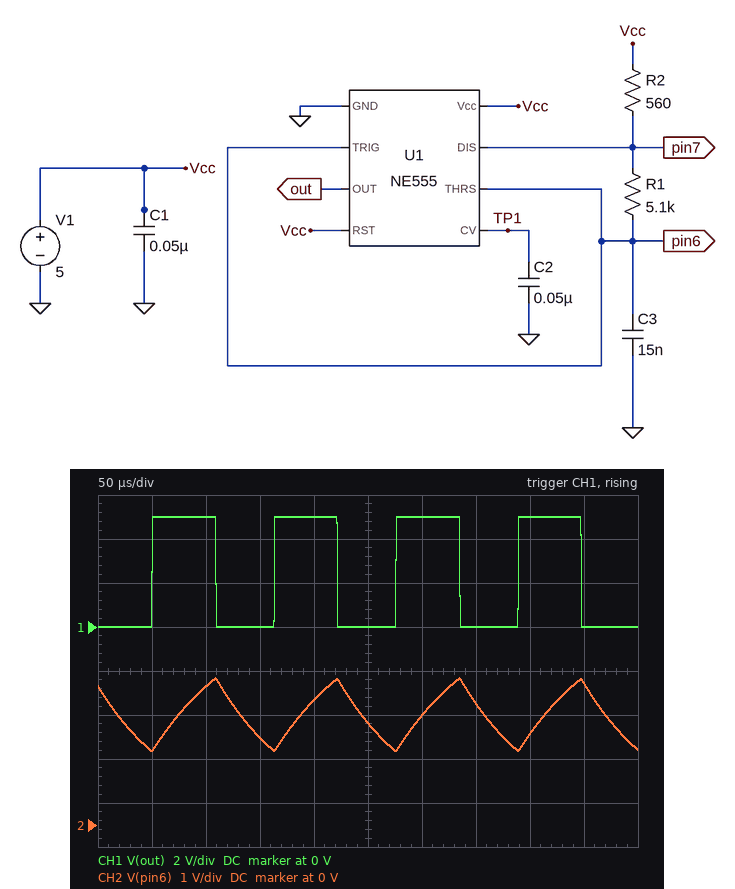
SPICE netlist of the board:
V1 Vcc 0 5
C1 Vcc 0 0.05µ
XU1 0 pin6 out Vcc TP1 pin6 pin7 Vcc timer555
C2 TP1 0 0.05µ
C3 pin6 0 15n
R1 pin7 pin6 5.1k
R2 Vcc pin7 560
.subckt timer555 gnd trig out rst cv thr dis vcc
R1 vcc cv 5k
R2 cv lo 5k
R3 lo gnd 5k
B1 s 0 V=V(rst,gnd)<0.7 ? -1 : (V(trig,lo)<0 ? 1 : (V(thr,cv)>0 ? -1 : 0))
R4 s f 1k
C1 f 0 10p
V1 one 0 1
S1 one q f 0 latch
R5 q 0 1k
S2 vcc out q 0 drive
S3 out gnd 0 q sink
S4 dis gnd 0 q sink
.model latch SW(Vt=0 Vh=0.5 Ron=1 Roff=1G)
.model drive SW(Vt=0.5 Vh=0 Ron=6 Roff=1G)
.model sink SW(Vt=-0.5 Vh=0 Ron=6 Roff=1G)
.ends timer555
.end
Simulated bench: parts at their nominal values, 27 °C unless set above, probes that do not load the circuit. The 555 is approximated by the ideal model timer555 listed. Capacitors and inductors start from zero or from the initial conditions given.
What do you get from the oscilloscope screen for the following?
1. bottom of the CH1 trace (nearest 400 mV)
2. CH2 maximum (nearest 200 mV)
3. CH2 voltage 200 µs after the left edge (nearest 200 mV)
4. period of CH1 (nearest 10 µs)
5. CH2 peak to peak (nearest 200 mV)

0 V
3.4 V
2.8 V
110 µs
1.6 V
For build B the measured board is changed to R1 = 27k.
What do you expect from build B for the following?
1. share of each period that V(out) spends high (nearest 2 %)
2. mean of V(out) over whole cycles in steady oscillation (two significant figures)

50 %
2.5 V
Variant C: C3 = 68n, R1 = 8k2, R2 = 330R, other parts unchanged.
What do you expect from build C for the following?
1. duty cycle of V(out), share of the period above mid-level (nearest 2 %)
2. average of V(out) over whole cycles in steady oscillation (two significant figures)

50 %
2.5 V
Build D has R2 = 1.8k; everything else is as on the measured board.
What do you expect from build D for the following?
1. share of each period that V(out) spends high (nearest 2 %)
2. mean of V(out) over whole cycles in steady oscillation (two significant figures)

58 %
2.9 V
